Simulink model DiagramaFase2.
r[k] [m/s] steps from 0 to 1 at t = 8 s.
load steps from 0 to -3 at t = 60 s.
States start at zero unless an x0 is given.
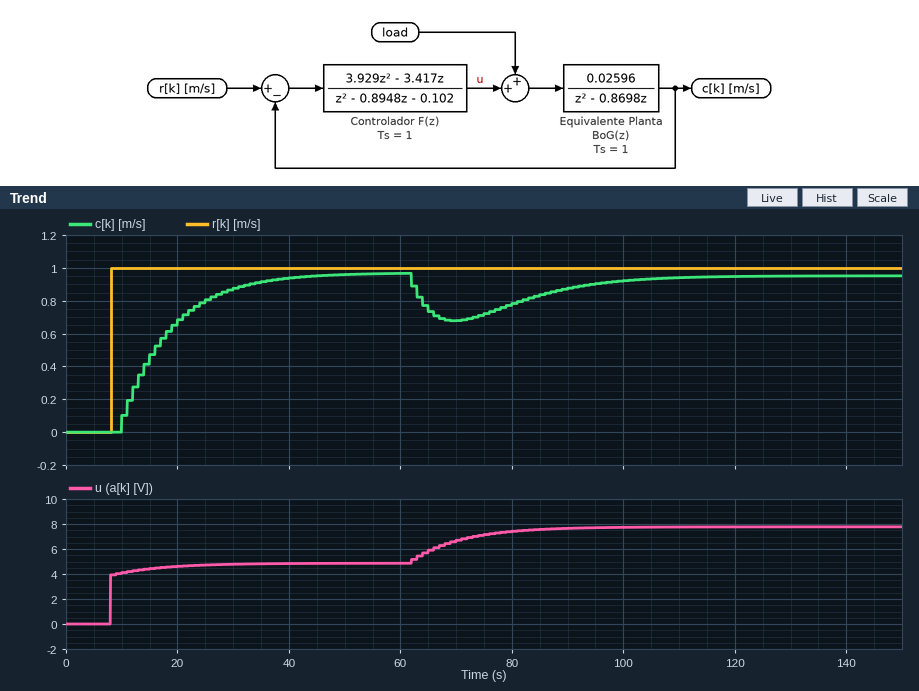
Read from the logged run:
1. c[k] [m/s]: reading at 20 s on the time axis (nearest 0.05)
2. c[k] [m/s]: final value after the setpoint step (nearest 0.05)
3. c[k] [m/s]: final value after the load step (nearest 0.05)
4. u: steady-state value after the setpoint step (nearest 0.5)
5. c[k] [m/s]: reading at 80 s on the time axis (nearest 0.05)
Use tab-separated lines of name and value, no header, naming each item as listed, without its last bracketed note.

c[k] [m/s]: reading at 20 s on the time axis	0.70
c[k] [m/s]: final value after the setpoint step	0.95
c[k] [m/s]: final value after the load step	0.95
u: steady-state value after the setpoint step	5.0
c[k] [m/s]: reading at 80 s on the time axis	0.80
